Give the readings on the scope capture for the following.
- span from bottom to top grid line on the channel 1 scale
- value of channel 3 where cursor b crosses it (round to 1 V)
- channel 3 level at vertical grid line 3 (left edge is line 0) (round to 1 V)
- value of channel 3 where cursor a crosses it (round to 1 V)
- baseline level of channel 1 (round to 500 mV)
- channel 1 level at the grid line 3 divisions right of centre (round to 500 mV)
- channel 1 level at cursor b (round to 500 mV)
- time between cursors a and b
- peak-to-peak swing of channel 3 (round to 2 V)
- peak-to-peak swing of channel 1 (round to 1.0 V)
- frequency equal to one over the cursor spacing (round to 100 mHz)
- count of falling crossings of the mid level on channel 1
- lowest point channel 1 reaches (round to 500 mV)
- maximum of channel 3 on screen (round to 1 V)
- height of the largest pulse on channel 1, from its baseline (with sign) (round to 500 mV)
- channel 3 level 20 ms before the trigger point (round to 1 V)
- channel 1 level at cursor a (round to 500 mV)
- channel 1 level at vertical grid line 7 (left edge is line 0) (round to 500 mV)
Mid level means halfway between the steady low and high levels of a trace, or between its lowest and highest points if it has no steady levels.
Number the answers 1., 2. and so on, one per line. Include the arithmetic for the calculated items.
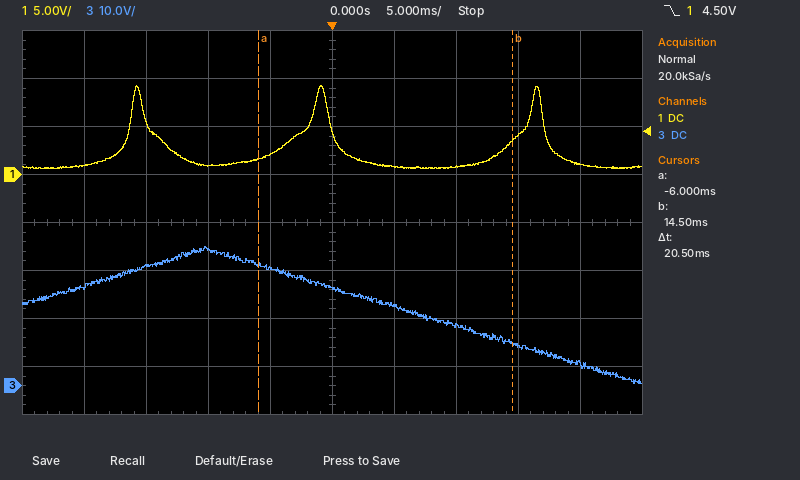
1. 40 V
2. 9 V
3. 28 V
4. 25 V
5. 1.0 V
6. 4.0 V
7. 3.5 V
8. 20.5 ms
9. 28 V
10. 9.0 V
11. 1 / 20.5 ms ≈ 48.8 Hz
12. 3
13. 500 mV
14. 29 V
15. +8.5 V
16. 21 V
17. 1.5 V
18. 1.0 V
